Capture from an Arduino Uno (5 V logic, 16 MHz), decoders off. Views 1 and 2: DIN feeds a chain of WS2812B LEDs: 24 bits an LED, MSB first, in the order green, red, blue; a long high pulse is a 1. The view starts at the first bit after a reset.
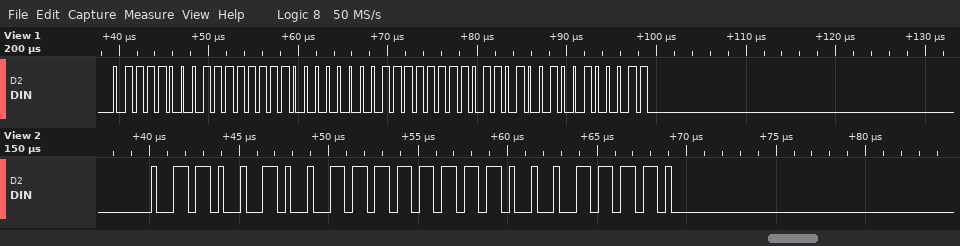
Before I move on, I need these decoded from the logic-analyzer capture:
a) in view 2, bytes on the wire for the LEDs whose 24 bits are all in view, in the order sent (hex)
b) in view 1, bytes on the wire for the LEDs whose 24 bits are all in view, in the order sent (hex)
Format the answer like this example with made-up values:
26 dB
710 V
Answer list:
64 FF 1E
78 FF 00 FF 69 23
